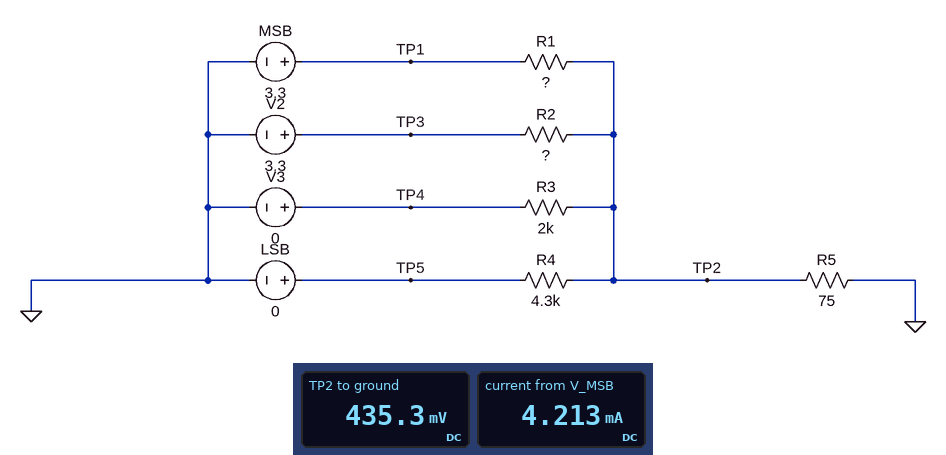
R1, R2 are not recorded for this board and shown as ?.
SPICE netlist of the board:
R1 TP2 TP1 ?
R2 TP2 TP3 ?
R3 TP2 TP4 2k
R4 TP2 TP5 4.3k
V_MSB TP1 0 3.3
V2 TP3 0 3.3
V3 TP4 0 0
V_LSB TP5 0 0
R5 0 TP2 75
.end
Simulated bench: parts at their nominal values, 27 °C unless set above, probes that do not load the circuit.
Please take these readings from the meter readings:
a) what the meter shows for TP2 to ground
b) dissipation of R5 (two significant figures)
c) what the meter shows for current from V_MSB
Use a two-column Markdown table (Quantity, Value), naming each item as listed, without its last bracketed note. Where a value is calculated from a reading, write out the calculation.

| Quantity | Value |
|---|---|
| what the meter shows for TP2 to ground | 435.3 mV |
| dissipation of R5 | (435.3 mV)^2 / 75 Ω = 2.5 mW |
| what the meter shows for current from V_MSB | 4.213 mA |
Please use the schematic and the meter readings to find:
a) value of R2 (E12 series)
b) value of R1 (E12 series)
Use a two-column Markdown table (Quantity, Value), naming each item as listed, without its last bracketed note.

| Quantity | Value |
|---|---|
| value of R2 | 1.5 kΩ |
| value of R1 | 680 Ω |
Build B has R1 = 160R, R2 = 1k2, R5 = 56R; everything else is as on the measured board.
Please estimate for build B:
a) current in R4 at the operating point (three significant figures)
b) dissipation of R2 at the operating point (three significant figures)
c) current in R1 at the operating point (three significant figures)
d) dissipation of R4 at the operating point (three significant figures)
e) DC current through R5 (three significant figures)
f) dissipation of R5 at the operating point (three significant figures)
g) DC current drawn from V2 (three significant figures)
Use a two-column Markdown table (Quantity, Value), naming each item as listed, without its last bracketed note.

| Quantity | Value |
|---|---|
| current in R4 at the operating point | 212 µA |
| dissipation of R2 at the operating point | 4.76 mW |
| current in R1 at the operating point | 14.9 mA |
| dissipation of R4 at the operating point | 193 µW |
| DC current through R5 | 16.3 mA |
| dissipation of R5 at the operating point | 14.8 mW |
| DC current drawn from V2 | 1.99 mA |
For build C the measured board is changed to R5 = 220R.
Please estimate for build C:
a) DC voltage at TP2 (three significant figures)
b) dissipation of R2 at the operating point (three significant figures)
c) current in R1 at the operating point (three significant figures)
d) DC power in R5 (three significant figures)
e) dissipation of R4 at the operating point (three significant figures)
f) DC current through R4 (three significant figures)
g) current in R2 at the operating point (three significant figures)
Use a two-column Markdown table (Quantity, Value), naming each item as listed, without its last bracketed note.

| Quantity | Value |
|---|---|
| DC voltage at TP2 | 951 mV |
| dissipation of R2 at the operating point | 3.68 mW |
| current in R1 at the operating point | 3.45 mA |
| DC power in R5 | 4.11 mW |
| dissipation of R4 at the operating point | 210 µW |
| DC current through R4 | 221 µA |
| current in R2 at the operating point | 1.57 mA |
